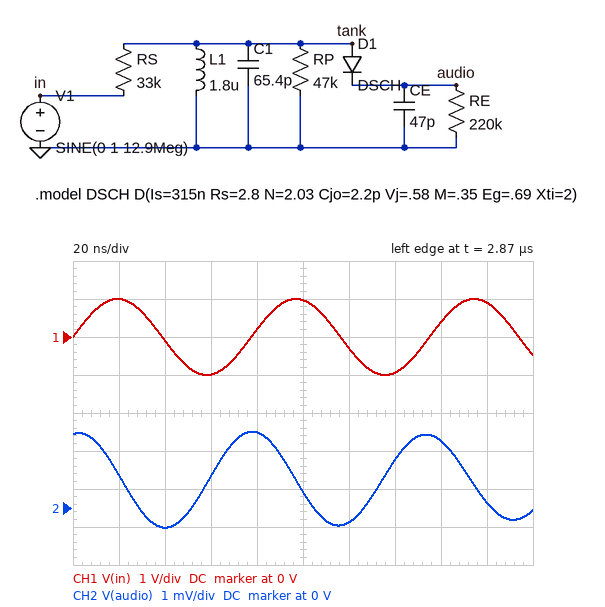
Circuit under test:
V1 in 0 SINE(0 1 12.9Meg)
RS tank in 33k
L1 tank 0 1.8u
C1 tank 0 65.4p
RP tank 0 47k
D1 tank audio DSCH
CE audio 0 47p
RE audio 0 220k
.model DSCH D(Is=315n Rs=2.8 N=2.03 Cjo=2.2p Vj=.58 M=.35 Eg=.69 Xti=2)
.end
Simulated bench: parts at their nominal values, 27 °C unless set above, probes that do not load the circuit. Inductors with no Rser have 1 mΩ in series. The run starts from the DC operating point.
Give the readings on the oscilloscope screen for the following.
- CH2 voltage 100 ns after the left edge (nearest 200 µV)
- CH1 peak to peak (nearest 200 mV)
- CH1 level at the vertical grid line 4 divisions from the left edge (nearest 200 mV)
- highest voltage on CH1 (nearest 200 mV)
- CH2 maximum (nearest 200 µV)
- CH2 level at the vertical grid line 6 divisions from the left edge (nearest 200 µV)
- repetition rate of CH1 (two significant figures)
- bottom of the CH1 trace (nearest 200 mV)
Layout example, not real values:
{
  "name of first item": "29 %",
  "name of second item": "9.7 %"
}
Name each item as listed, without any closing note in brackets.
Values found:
{
  "CH2 voltage 100 ns after the left edge": "400 µV",
  "CH1 peak to peak": "2.0 V",
  "CH1 level at the vertical grid line 4 divisions from the left edge": "200 mV",
  "highest voltage on CH1": "1.0 V",
  "CH2 maximum": "2.0 mV",
  "CH2 level at the vertical grid line 6 divisions from the left edge": "-400 µV",
  "repetition rate of CH1": "13 MHz",
  "bottom of the CH1 trace": "-1.0 V"
}
